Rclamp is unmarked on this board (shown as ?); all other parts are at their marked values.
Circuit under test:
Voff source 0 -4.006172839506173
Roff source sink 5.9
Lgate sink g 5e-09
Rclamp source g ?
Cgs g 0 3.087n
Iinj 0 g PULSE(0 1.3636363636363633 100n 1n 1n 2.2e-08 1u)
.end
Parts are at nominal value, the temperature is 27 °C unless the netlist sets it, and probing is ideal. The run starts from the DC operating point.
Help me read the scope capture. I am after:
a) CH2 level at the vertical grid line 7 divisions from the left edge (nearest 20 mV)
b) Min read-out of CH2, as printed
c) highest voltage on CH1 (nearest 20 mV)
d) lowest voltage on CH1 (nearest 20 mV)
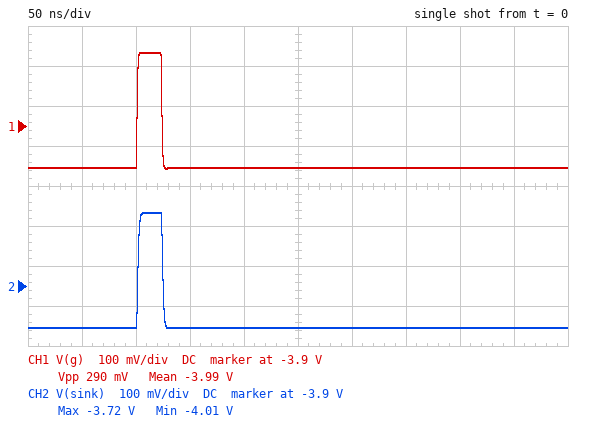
-4.00 V
-4.01 V
-3.72 V
-4.00 V
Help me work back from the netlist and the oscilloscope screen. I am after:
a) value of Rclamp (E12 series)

0.22 Ω
